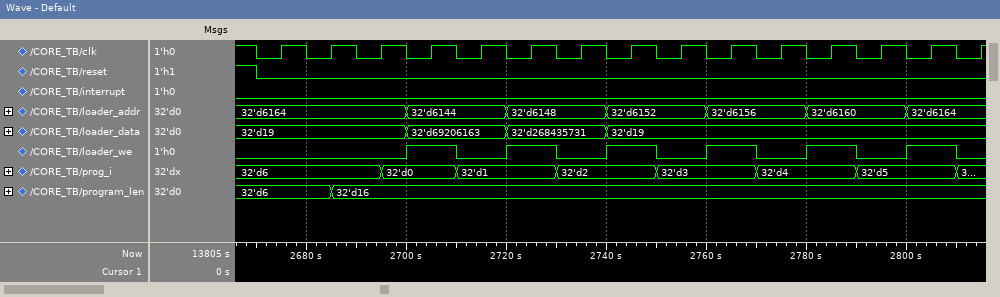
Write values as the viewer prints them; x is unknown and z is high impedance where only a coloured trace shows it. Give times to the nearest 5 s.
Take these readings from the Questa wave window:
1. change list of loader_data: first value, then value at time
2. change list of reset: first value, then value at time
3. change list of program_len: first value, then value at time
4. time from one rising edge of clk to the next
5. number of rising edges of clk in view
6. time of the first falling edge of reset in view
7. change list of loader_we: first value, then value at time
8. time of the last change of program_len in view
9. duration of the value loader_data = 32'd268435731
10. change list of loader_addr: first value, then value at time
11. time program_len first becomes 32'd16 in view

32'd19, 32'd69206163 at 2700 s, 32'd268435731 at 2720 s, 32'd19 at 2740 s
1, 0 at 2670 s
32'd6, 32'd16 at 2685 s
10 s
15
2670 s
0, 1 at 2700 s, 0 at 2710 s, 1 at 2720 s, 0 at 2730 s, 1 at 2740 s, 0 at 2750 s, 1 at 2760 s, 0 at 2770 s, 1 at 2780 s, 0 at 2790 s, 1 at 2800 s, 0 at 2810 s
2685 s
20 s
32'd6164, 32'd6144 at 2700 s, 32'd6148 at 2720 s, 32'd6152 at 2740 s, 32'd6156 at 2760 s, 32'd6160 at 2780 s, 32'd6164 at 2800 s
2685 s
